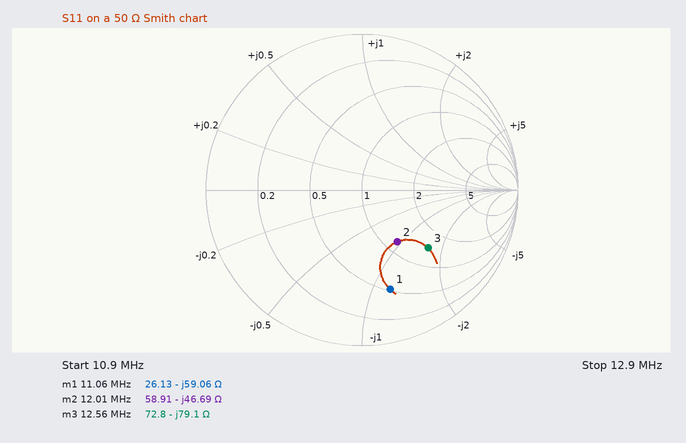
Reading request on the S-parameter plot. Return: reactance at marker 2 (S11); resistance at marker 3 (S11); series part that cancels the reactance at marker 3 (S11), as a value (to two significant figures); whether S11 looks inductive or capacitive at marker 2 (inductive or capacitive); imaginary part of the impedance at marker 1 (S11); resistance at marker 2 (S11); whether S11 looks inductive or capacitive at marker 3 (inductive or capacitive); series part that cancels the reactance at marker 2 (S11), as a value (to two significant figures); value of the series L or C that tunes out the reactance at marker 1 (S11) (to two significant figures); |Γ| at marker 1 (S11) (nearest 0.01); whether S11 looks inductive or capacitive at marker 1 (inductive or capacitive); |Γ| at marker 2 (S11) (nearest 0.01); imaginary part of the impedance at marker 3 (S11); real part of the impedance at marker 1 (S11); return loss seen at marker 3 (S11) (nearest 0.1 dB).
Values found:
-46.69 Ω
72.8 Ω
1.0 µH
capacitive
-59.06 Ω
58.91 Ω
capacitive
620 nH
850 nH
0.66
capacitive
0.40
-79.1 Ω
26.13 Ω
5.0 dB
